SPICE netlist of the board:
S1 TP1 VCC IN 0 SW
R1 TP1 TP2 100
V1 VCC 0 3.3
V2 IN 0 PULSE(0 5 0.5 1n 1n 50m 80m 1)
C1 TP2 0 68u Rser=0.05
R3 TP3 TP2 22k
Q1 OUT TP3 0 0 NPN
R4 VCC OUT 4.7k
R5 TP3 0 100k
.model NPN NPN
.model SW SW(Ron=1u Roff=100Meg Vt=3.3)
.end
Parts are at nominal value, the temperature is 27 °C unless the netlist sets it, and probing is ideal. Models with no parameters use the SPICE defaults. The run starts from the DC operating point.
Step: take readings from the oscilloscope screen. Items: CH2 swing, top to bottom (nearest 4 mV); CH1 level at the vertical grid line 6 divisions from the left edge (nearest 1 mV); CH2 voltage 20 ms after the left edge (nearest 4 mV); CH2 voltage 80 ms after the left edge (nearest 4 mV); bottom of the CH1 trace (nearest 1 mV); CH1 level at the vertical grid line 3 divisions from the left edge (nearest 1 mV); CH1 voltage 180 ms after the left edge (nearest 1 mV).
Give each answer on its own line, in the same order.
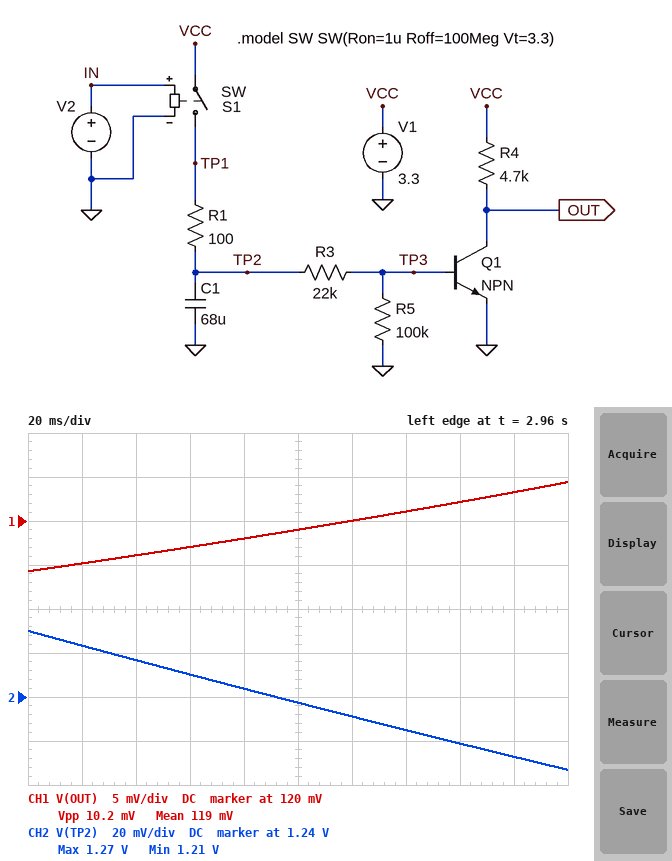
64 mV
120 mV
1.264 V
1.244 V
114 mV
117 mV
123 mV
